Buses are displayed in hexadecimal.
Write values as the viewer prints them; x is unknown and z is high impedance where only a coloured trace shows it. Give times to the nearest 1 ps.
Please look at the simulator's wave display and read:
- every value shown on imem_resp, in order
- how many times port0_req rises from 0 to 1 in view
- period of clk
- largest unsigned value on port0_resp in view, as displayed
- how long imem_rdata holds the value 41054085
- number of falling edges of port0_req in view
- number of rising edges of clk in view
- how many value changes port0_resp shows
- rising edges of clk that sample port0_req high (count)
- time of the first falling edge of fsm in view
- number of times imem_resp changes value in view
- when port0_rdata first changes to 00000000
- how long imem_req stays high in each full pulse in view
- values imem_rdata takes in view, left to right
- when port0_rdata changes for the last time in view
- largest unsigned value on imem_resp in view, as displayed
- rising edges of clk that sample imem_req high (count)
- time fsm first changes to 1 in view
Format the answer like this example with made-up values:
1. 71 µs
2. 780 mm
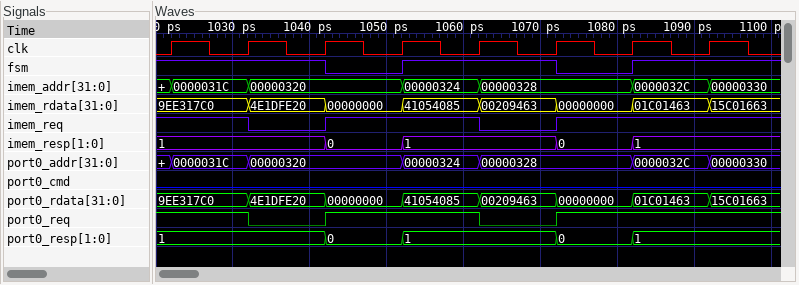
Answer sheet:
1. 1, 0, 1, 0, 1
2. 2
3. 10 ps
4. 1
5. 10 ps
6. 2
7. 8
8. 4
9. 6
10. 1042 ps
11. 4
12. 1042 ps
13. 20 ps
14. 9EE317C0, 4E1DFE20, 00000000, 41054085, 00209463, 00000000, 01C01463, 15C01663
15. 1092 ps
16. 1
17. 6
18. 1052 ps
